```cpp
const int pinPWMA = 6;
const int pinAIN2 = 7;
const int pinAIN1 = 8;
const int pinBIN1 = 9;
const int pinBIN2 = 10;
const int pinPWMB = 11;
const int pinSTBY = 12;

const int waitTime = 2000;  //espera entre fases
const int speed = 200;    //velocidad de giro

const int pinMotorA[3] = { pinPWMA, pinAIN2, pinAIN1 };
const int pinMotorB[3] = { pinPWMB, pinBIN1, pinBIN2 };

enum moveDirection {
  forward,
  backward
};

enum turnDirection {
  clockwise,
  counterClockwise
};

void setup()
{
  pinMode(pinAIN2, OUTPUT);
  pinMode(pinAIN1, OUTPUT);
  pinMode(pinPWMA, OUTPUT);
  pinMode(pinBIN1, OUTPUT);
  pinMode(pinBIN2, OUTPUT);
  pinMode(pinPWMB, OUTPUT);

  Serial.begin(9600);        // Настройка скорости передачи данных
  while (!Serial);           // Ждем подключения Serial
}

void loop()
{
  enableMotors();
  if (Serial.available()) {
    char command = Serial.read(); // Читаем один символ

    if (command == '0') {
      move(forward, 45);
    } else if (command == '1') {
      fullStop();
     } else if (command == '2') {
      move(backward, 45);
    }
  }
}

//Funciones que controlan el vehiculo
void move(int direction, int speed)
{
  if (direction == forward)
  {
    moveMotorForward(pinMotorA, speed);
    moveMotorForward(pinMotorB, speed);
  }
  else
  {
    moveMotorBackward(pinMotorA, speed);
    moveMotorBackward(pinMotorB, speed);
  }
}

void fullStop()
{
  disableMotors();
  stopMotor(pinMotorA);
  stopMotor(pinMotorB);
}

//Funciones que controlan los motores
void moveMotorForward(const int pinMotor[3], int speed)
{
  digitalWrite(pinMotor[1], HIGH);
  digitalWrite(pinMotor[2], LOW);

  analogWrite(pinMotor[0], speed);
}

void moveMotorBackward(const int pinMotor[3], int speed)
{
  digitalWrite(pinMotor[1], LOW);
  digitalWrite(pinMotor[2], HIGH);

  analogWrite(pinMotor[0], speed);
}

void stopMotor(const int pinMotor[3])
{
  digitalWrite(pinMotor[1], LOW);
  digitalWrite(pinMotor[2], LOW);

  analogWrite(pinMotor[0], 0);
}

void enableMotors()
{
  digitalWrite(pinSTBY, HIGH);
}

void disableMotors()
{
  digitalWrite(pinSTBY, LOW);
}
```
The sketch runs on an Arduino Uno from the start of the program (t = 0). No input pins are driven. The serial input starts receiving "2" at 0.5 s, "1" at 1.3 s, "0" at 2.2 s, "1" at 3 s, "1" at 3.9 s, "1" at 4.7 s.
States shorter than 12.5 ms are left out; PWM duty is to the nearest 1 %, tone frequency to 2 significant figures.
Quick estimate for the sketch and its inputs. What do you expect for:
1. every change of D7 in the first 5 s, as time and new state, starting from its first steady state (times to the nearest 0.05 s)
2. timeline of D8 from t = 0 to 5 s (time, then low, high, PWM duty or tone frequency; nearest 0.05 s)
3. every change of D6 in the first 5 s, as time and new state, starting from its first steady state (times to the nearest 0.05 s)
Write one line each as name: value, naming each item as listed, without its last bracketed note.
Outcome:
every change of D7 in the first 5 s, as time and new state, starting from its first steady state: 0 s low; 2.2 s high; 3 s low
timeline of D8 from t = 0 to 5 s: 0 s low; 0.5 s high; 1.3 s low
every change of D6 in the first 5 s, as time and new state, starting from its first steady state: 0 s low; 0.5 s PWM 18 %; 1.3 s low; 2.2 s PWM 18 %; 3 s low
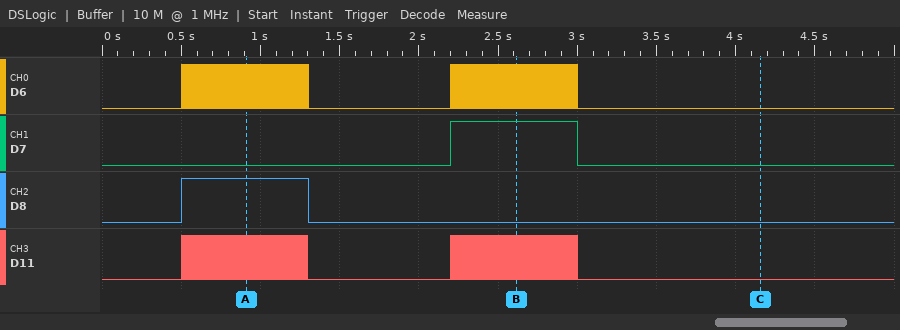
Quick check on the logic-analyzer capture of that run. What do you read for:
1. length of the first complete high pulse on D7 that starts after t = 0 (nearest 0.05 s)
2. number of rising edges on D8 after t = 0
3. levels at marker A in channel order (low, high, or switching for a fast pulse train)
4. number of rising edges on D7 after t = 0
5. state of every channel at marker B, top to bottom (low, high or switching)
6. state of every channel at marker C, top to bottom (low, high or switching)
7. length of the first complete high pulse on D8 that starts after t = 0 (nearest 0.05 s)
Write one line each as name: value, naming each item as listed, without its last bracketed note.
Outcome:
length of the first complete high pulse on D7 that starts after t = 0: 0.80 s
number of rising edges on D8 after t = 0: 1
levels at marker A in channel order: D6 switching, D7 low, D8 high, D11 switching
number of rising edges on D7 after t = 0: 1
state of every channel at marker B, top to bottom: D6 switching, D7 high, D8 low, D11 switching
state of every channel at marker C, top to bottom: D6 low, D7 low, D8 low, D11 low
length of the first complete high pulse on D8 that starts after t = 0: 0.80 s
